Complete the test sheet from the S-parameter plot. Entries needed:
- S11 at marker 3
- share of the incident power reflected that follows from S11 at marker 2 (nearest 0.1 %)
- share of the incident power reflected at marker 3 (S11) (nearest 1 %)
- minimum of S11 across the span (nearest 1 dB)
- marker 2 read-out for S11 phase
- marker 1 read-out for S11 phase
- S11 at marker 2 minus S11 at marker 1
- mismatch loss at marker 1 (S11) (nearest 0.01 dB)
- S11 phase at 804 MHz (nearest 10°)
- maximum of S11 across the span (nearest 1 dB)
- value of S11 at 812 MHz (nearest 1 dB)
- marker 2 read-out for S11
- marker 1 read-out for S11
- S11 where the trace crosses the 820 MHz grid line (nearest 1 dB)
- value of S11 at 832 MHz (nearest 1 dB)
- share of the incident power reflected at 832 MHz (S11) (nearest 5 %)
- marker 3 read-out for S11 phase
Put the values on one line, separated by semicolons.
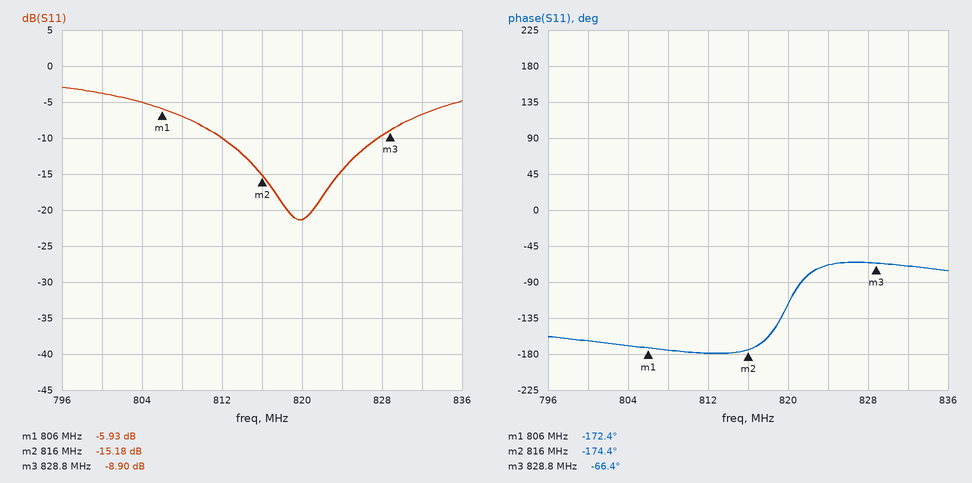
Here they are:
-8.90 dB; 3.0 %; 13 %; -21 dB; -174.4°; -172.4°; -9.25 dB; 1.28 dB; -170°; -3 dB; -10 dB; -15.18 dB; -5.93 dB; -21 dB; -7 dB; 20 %; -66.4°
